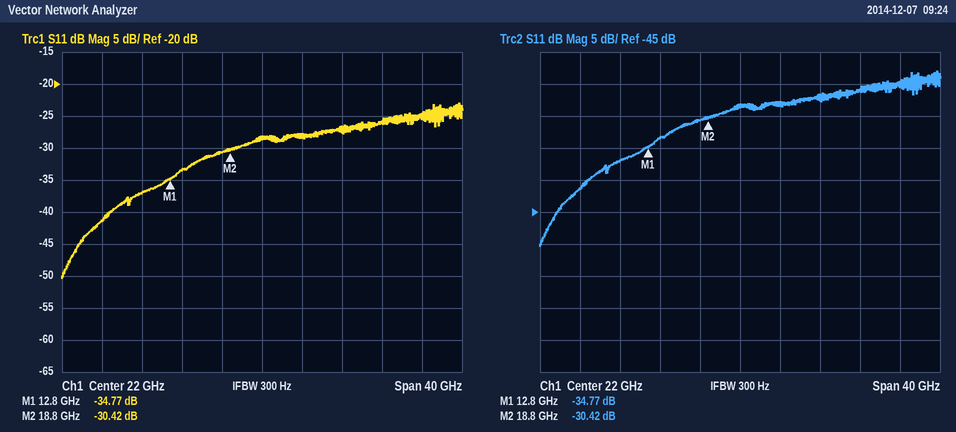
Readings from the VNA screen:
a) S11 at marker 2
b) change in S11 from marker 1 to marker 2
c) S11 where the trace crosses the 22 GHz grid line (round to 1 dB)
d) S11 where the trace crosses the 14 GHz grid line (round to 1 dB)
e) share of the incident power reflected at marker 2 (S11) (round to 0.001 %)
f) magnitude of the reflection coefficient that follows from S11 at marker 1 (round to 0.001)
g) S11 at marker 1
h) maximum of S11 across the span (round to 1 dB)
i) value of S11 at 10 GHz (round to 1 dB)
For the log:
-30.42 dB
4.35 dB
-28 dB
-33 dB
0.091 %
0.018
-34.77 dB
-23 dB
-37 dB
